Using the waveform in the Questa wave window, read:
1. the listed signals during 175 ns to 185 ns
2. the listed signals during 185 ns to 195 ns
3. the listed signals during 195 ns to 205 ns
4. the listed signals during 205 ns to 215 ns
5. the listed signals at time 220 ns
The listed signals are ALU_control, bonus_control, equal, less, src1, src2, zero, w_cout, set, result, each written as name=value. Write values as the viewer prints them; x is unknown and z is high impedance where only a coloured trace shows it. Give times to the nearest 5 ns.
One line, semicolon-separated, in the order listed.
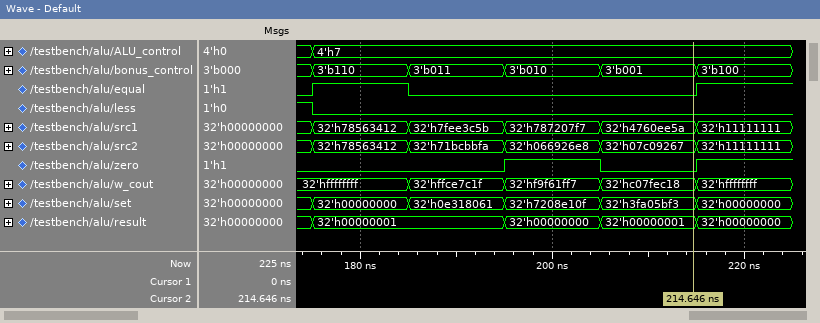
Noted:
ALU_control=4'h7, bonus_control=3'b110, equal=1, less=0, src1=32'h78563412, src2=32'h78563412, zero=0, w_cout=32'hffffffff, set=32'h00000000, result=32'h00000001; ALU_control=4'h7, bonus_control=3'b011, equal=0, less=0, src1=32'h7fee3c5b, src2=32'h71bcbbfa, zero=0, w_cout=32'hffce7c1f, set=32'h0e318061, result=32'h00000001; ALU_control=4'h7, bonus_control=3'b010, equal=0, less=0, src1=32'h787207f7, src2=32'h066926e8, zero=1, w_cout=32'hf9f61ff7, set=32'h7208e10f, result=32'h00000000; ALU_control=4'h7, bonus_control=3'b001, equal=0, less=0, src1=32'h4760ee5a, src2=32'h07c09267, zero=0, w_cout=32'hc07fec18, set=32'h3fa05bf3, result=32'h00000001; ALU_control=4'h7, bonus_control=3'b100, equal=1, less=0, src1=32'h11111111, src2=32'h11111111, zero=1, w_cout=32'hffffffff, set=32'h00000000, result=32'h00000000
